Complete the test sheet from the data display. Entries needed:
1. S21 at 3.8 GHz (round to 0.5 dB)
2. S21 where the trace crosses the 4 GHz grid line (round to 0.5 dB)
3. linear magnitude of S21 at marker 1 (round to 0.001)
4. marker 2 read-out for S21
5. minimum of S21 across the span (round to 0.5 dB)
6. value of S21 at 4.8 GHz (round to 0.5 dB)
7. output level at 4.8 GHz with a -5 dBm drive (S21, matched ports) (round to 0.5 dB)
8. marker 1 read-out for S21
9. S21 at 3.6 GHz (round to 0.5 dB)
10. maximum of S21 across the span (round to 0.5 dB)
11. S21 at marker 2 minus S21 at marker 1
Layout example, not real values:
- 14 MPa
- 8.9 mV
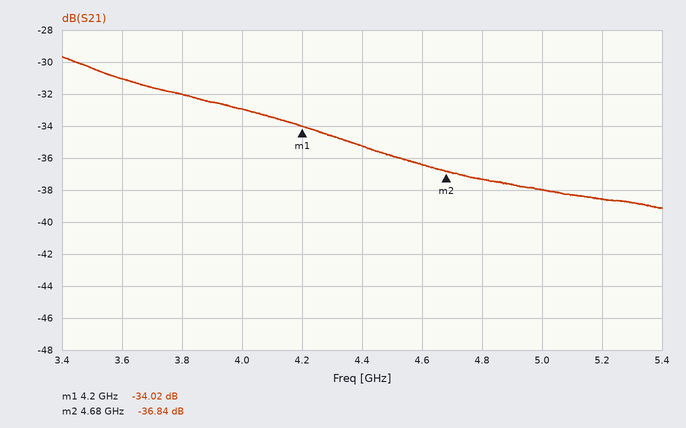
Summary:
- -32.0 dB
- -33.0 dB
- 0.020
- -36.84 dB
- -39.0 dB
- -37.5 dB
- -42.5 dBm
- -34.02 dB
- -31.0 dB
- -29.5 dB
- -2.82 dB
